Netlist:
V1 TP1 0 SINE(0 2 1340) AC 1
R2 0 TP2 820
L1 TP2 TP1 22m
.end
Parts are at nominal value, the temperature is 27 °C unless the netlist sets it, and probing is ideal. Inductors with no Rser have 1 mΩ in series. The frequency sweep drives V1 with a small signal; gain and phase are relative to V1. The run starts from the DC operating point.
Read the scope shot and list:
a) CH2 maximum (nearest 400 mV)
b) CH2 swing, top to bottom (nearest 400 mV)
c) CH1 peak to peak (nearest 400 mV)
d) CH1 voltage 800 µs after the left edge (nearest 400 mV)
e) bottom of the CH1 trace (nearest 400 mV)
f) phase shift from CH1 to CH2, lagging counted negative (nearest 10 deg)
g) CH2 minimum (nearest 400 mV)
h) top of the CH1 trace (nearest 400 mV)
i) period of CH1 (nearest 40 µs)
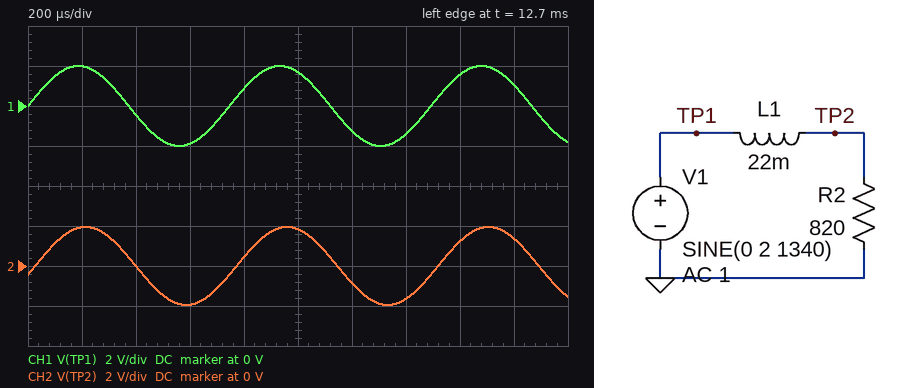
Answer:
2.0 V
4.0 V
4.0 V
800 mV
-2.0 V
-10 deg
-2.0 V
2.0 V
760 µs
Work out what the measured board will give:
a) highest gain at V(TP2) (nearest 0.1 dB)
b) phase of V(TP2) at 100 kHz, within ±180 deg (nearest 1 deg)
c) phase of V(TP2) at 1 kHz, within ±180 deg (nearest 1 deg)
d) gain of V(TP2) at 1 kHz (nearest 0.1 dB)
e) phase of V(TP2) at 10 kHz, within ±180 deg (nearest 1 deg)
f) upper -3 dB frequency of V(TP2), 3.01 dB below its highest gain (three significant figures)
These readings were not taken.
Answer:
0 dB
-87 deg
-10 deg
-0.1 dB
-59 deg
5.93 kHz
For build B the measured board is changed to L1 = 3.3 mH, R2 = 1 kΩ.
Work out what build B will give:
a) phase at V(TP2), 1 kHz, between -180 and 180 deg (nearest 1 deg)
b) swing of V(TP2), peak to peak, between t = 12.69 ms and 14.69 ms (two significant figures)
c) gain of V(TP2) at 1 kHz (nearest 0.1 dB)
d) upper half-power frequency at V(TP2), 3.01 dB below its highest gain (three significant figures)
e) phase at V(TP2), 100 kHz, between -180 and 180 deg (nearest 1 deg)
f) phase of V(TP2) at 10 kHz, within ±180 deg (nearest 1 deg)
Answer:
-1 deg
4.0 V
0 dB
48.2 kHz
-64 deg
-12 deg
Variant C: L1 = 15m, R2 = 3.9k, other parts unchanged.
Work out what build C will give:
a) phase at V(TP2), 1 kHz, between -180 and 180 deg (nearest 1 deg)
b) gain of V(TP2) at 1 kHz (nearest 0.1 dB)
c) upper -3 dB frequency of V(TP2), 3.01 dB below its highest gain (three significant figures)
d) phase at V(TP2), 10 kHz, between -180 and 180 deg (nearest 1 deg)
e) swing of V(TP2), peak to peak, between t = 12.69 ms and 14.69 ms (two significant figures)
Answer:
-1 deg
0 dB
41.4 kHz
-14 deg
4.0 V
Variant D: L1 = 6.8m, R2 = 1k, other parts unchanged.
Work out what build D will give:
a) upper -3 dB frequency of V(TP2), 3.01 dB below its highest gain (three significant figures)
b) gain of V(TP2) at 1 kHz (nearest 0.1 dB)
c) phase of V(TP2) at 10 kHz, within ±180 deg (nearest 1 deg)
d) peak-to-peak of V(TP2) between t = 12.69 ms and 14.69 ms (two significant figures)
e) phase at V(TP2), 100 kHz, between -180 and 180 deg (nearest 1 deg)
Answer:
23.4 kHz
0 dB
-23 deg
4.0 V
-77 deg
